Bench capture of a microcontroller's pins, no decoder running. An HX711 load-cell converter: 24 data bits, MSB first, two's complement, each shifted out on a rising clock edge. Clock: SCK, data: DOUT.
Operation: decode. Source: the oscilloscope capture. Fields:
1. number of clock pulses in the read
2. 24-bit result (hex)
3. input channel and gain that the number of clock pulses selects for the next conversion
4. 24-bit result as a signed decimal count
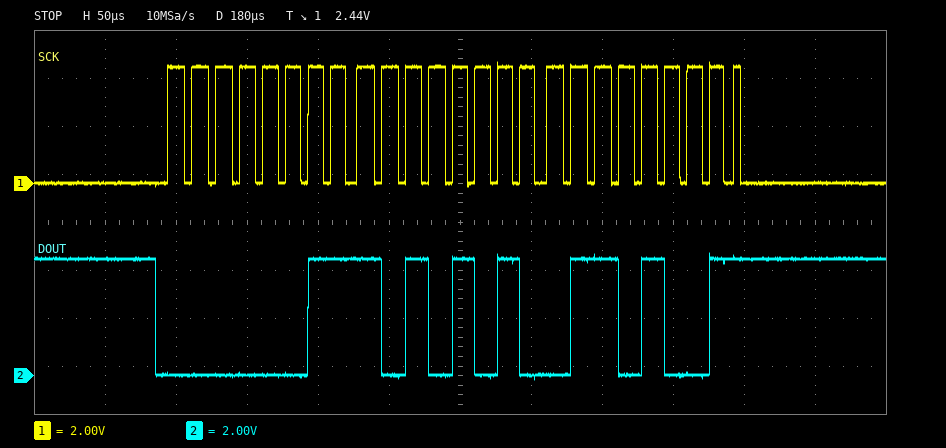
25
0x03AA69
channel A, gain 128
240233
